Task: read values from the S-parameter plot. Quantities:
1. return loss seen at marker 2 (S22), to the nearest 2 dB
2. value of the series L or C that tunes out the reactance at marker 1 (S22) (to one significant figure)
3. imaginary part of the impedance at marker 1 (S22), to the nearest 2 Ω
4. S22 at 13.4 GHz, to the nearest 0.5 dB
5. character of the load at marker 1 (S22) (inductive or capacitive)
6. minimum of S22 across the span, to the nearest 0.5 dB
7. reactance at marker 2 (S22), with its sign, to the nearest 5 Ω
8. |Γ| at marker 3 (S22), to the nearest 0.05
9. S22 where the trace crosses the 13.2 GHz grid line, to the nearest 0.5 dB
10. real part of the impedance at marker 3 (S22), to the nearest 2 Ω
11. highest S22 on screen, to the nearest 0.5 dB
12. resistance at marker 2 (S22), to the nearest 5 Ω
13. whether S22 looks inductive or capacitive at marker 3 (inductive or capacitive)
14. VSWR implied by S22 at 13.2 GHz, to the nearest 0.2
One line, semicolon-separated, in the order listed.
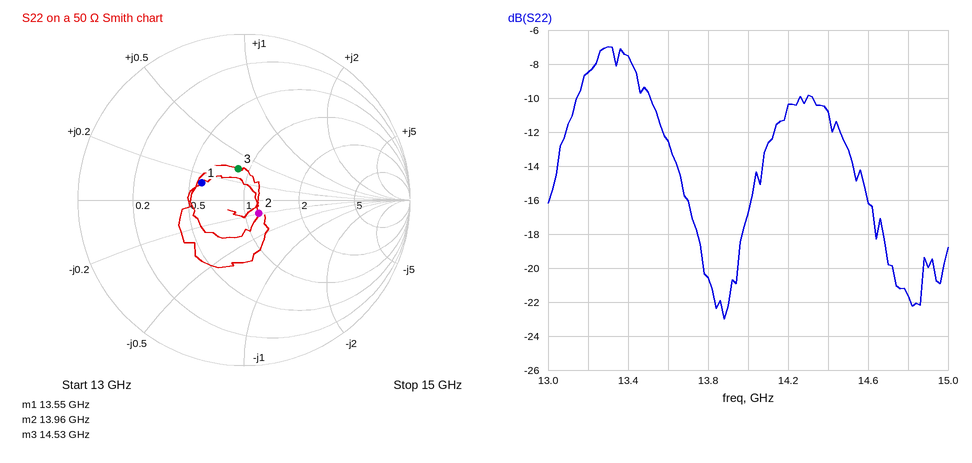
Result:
18 dB; 2 pF; +6 Ω; -7.5 dB; inductive; -23.0 dB; -10 Ω; 0.20; -8.5 dB; 44 Ω; -7.0 dB; 60 Ω; inductive; 2.2
